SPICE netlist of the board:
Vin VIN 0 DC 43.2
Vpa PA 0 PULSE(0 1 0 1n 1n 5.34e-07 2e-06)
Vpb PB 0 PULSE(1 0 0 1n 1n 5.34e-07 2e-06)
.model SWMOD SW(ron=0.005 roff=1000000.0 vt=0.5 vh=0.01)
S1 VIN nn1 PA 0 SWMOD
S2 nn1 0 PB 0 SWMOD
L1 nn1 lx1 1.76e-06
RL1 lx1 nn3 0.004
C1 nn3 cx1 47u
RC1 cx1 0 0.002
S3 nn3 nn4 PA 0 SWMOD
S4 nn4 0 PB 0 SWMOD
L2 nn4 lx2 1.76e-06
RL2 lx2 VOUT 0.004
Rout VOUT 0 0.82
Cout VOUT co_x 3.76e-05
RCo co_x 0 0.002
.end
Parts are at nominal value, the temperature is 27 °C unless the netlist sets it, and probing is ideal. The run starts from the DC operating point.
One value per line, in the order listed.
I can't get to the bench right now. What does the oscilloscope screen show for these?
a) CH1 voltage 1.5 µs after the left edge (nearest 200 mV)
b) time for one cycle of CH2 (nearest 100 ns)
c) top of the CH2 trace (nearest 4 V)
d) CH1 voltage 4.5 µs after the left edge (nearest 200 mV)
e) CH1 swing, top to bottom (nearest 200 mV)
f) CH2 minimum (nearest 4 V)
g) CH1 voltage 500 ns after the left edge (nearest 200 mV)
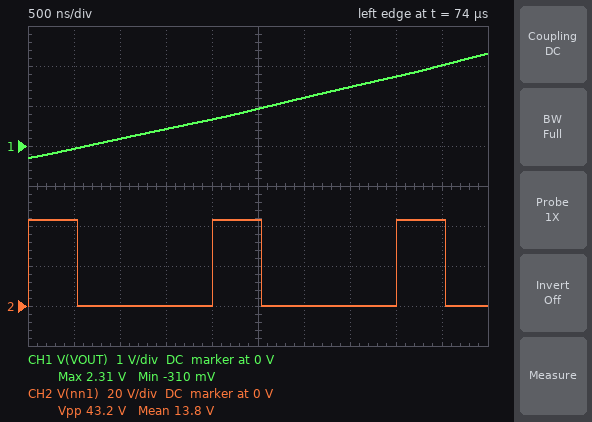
400 mV
2.0 µs
44 V
2.0 V
2.6 V
0 V
0 V
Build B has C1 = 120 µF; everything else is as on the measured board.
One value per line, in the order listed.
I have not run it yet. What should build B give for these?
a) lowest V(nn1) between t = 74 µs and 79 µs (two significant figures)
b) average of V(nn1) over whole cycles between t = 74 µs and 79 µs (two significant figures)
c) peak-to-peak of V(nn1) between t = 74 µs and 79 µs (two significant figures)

250 mV
12 V
43 V
